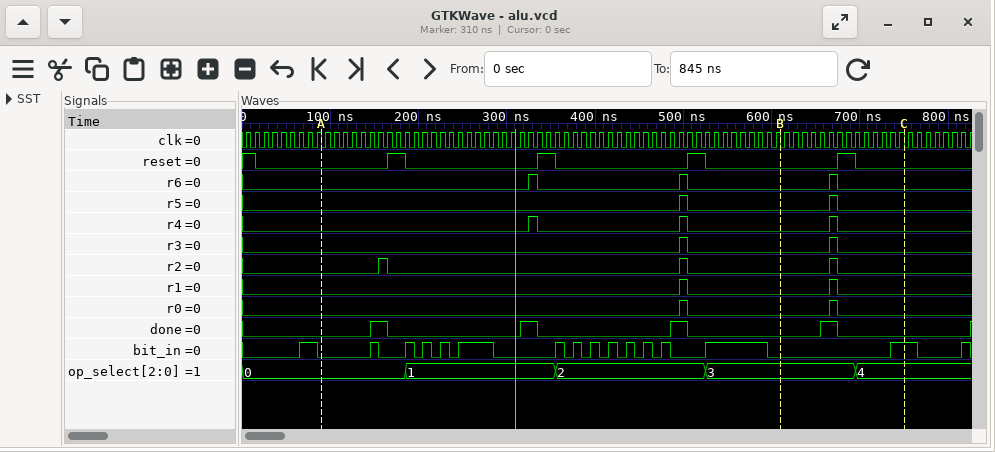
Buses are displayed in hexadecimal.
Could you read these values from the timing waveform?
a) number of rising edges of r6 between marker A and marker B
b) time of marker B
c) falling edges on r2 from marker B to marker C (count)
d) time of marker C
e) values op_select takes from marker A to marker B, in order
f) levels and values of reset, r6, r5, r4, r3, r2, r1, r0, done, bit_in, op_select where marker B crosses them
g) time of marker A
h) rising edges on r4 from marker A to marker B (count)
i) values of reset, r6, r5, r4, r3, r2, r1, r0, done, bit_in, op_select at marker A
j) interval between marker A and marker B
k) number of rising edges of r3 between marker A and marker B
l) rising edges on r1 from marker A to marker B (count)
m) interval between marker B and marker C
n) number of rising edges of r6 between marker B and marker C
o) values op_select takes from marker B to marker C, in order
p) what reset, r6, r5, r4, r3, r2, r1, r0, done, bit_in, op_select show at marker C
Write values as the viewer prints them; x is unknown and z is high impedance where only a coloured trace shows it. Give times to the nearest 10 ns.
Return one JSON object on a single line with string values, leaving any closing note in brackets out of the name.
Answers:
{"number of rising edges of r6 between marker A and marker B": "2", "time of marker B": "610 ns", "falling edges on r2 from marker B to marker C": "1", "time of marker C": "750 ns", "values op_select takes from marker A to marker B, in order": "0, 1, 2, 3", "levels and values of reset, r6, r5, r4, r3, r2, r1, r0, done, bit_in, op_select where marker B crosses them": "reset=0, r6=0, r5=0, r4=0, r3=0, r2=0, r1=0, r0=0, done=0, bit_in=0, op_select=3", "time of marker A": "90 ns", "rising edges on r4 from marker A to marker B": "2", "values of reset, r6, r5, r4, r3, r2, r1, r0, done, bit_in, op_select at marker A": "reset=0, r6=0, r5=0, r4=0, r3=0, r2=0, r1=0, r0=0, done=0, bit_in=0, op_select=0", "interval between marker A and marker B": "520 ns", "number of rising edges of r3 between marker A and marker B": "1", "rising edges on r1 from marker A to marker B": "1", "interval between marker B and marker C": "140 ns", "number of rising edges of r6 between marker B and marker C": "1", "values op_select takes from marker B to marker C, in order": "3, 4", "what reset, r6, r5, r4, r3, r2, r1, r0, done, bit_in, op_select show at marker C": "reset=0, r6=0, r5=0, r4=0, r3=0, r2=0, r1=0, r0=0, done=0, bit_in=1, op_select=4"}
